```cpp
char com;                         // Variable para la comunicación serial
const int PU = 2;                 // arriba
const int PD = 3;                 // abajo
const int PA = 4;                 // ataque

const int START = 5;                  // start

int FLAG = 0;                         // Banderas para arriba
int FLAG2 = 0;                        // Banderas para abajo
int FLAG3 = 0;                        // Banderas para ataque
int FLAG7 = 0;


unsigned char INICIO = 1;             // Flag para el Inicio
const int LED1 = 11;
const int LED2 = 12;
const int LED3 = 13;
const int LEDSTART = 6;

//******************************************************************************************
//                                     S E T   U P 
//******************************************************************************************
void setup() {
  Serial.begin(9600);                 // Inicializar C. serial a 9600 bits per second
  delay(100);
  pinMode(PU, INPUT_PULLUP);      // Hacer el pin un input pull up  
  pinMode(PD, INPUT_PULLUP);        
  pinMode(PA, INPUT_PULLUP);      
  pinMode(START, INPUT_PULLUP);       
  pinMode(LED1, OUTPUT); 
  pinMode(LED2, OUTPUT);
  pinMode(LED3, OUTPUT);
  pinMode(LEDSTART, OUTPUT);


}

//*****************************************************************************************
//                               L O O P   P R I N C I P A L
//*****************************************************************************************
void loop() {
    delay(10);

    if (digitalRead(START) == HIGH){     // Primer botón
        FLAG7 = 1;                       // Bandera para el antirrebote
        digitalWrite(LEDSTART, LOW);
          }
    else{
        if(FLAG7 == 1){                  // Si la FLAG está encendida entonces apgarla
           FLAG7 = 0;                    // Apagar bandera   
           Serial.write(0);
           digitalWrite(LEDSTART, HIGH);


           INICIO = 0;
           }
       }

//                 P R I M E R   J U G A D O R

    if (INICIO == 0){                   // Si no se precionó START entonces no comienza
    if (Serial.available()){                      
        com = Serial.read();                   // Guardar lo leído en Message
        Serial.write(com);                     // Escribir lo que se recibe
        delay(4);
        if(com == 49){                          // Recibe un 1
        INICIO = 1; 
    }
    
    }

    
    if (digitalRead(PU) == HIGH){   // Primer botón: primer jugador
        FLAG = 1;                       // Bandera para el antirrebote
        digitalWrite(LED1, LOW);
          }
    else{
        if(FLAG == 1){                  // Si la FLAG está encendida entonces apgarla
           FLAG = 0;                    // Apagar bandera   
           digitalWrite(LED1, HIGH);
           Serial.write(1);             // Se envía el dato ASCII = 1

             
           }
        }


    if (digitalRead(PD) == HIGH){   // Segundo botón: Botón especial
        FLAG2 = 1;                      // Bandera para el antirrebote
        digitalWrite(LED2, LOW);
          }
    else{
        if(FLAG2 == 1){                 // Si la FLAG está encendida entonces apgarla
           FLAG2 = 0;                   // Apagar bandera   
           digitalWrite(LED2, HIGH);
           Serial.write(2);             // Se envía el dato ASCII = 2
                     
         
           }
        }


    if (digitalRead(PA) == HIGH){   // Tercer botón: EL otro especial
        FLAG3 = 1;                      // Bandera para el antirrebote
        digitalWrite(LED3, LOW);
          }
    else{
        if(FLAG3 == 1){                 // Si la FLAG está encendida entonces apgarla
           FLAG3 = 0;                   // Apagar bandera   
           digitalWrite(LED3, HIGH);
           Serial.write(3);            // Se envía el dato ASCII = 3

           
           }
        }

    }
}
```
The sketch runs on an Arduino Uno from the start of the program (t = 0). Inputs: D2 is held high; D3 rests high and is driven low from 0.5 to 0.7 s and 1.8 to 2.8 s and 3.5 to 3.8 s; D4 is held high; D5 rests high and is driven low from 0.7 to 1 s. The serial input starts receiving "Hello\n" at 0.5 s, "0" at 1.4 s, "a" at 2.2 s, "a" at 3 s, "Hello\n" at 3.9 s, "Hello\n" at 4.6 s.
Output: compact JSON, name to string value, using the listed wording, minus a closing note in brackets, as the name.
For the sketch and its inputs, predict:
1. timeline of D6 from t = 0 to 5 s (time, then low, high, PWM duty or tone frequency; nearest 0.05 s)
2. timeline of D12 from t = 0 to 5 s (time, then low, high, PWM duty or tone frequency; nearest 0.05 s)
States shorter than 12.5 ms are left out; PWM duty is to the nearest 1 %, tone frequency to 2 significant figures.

{"timeline of D6 from t = 0 to 5 s": "0.1 s low; 0.7 s high; 1 s low", "timeline of D12 from t = 0 to 5 s": "0.1 s low; 1.8 s high; 2.8 s low; 3.5 s high; 3.8 s low"}
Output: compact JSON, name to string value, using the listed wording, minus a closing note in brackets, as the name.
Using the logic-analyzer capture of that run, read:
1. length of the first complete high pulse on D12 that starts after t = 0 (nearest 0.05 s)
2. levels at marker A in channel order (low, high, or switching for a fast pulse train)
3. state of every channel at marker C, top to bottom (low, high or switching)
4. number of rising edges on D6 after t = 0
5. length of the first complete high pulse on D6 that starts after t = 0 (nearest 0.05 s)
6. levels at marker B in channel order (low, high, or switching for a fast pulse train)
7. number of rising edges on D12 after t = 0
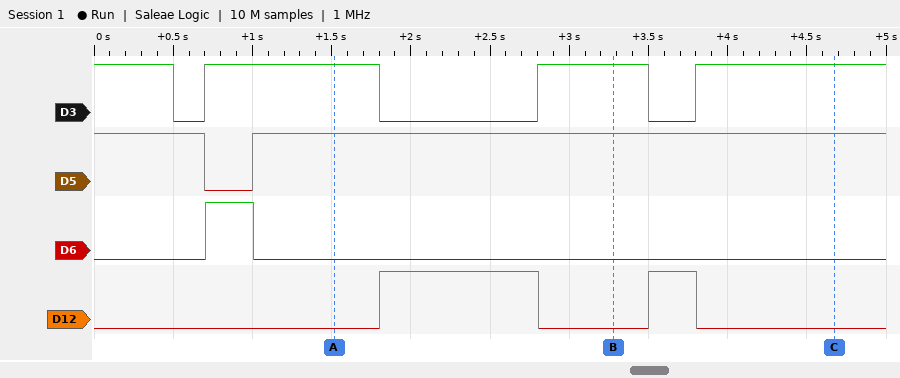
{"length of the first complete high pulse on D12 that starts after t = 0": "1.00 s", "levels at marker A in channel order": "D3 high, D5 high, D6 low, D12 low", "state of every channel at marker C, top to bottom": "D3 high, D5 high, D6 low, D12 low", "number of rising edges on D6 after t = 0": "1", "length of the first complete high pulse on D6 that starts after t = 0": "0.30 s", "levels at marker B in channel order": "D3 high, D5 high, D6 low, D12 low", "number of rising edges on D12 after t = 0": "2"}
